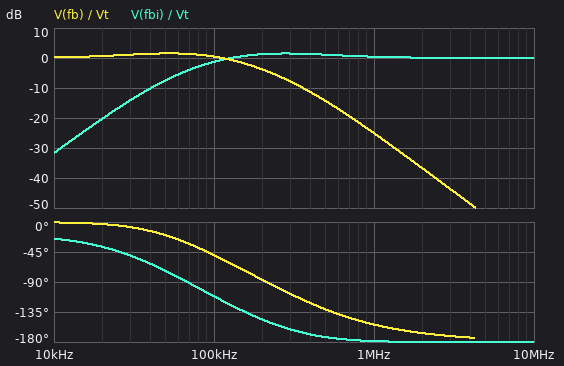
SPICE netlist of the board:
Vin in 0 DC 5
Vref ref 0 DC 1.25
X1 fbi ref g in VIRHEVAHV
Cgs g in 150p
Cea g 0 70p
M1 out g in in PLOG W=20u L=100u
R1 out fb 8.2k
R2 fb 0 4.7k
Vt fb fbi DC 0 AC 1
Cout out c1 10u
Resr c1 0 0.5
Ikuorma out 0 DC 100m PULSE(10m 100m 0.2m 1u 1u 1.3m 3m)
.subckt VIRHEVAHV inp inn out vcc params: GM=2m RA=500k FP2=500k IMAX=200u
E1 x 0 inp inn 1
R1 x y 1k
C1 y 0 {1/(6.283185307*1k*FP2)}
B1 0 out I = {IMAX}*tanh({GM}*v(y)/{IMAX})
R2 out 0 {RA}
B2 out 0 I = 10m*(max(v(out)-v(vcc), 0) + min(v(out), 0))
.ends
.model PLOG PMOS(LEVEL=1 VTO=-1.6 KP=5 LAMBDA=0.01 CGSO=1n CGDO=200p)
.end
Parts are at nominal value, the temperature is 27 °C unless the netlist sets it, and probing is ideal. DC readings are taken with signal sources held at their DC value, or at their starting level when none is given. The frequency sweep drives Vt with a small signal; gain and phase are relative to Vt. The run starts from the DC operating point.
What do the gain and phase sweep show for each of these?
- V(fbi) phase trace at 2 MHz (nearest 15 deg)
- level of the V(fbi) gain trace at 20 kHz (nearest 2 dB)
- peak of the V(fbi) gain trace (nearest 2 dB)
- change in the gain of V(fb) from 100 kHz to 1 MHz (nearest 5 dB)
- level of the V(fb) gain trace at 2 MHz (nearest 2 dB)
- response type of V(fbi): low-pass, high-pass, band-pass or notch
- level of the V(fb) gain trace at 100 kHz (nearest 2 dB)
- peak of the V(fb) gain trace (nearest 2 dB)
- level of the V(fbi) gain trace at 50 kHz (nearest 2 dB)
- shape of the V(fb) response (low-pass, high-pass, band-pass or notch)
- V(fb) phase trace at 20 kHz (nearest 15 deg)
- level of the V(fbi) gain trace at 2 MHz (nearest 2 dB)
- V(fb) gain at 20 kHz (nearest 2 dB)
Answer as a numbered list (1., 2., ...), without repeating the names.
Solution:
1. -180 deg
2. -20 dB
3. 2 dB
4. -25 dB
5. -36 dB
6. high-pass
7. 0 dB
8. 2 dB
9. -8 dB
10. low-pass
11. 0 deg
12. 0 dB
13. 0 dB
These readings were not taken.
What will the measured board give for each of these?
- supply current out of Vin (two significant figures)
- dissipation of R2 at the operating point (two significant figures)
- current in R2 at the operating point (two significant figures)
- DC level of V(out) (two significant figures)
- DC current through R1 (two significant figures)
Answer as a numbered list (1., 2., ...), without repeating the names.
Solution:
1. 100 mA
2. 330 µW
3. 270 µA
4. 3.4 V
5. 270 µA
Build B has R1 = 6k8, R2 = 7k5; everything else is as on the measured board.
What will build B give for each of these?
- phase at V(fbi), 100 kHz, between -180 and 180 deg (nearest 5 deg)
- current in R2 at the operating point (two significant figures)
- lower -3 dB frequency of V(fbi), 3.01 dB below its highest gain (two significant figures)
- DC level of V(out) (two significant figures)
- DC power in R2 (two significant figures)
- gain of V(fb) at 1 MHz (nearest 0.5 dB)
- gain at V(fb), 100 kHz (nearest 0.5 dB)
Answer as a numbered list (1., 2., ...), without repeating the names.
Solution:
1. -95 deg
2. 170 µA
3. 140 kHz
4. 2.4 V
5. 210 µW
6. -21.5 dB
7. 1.0 dB
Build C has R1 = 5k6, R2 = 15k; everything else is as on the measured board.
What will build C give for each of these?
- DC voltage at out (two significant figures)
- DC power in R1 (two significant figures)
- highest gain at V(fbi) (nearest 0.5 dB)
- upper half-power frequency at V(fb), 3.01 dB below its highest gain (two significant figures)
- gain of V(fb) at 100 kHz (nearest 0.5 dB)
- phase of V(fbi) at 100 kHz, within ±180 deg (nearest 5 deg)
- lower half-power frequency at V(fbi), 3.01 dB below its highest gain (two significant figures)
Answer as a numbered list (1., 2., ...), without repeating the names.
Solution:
1. 1.7 V
2. 39 µW
3. 2.5 dB
4. 320 kHz
5. 1.0 dB
6. -85 deg
7. 200 kHz
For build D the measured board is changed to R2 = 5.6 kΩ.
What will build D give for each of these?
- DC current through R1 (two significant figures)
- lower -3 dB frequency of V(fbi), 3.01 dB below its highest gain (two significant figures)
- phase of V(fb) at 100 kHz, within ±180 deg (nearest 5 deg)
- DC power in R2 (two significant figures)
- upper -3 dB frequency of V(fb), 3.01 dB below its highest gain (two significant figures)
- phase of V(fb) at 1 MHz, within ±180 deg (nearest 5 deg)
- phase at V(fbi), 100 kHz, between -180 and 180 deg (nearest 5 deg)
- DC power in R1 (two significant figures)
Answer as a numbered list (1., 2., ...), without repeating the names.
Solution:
1. 220 µA
2. 110 kHz
3. -45 deg
4. 280 µW
5. 170 kHz
6. -155 deg
7. -105 deg
8. 410 µW
